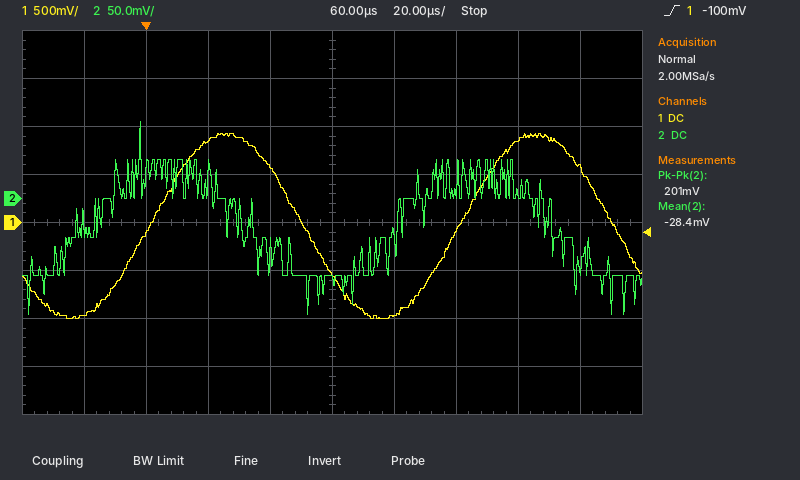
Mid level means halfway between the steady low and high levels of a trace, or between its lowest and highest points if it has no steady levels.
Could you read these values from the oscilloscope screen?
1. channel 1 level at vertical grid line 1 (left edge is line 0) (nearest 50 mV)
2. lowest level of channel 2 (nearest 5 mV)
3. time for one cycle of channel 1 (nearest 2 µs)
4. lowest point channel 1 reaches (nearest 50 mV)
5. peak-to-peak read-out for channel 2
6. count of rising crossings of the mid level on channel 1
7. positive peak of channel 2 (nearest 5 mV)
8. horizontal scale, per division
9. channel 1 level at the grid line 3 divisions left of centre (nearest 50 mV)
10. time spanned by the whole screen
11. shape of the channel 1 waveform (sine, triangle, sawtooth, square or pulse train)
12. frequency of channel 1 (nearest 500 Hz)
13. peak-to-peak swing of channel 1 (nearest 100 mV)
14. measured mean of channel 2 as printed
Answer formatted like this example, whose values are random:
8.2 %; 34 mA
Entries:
-950 mV; -120 mV; 100 µs; -1.00 V; 201 mV; 2; 80 mV; 20 µs; -100 mV; 200 µs; sine; 10.0 kHz; 1.90 V; -28.4 mV
